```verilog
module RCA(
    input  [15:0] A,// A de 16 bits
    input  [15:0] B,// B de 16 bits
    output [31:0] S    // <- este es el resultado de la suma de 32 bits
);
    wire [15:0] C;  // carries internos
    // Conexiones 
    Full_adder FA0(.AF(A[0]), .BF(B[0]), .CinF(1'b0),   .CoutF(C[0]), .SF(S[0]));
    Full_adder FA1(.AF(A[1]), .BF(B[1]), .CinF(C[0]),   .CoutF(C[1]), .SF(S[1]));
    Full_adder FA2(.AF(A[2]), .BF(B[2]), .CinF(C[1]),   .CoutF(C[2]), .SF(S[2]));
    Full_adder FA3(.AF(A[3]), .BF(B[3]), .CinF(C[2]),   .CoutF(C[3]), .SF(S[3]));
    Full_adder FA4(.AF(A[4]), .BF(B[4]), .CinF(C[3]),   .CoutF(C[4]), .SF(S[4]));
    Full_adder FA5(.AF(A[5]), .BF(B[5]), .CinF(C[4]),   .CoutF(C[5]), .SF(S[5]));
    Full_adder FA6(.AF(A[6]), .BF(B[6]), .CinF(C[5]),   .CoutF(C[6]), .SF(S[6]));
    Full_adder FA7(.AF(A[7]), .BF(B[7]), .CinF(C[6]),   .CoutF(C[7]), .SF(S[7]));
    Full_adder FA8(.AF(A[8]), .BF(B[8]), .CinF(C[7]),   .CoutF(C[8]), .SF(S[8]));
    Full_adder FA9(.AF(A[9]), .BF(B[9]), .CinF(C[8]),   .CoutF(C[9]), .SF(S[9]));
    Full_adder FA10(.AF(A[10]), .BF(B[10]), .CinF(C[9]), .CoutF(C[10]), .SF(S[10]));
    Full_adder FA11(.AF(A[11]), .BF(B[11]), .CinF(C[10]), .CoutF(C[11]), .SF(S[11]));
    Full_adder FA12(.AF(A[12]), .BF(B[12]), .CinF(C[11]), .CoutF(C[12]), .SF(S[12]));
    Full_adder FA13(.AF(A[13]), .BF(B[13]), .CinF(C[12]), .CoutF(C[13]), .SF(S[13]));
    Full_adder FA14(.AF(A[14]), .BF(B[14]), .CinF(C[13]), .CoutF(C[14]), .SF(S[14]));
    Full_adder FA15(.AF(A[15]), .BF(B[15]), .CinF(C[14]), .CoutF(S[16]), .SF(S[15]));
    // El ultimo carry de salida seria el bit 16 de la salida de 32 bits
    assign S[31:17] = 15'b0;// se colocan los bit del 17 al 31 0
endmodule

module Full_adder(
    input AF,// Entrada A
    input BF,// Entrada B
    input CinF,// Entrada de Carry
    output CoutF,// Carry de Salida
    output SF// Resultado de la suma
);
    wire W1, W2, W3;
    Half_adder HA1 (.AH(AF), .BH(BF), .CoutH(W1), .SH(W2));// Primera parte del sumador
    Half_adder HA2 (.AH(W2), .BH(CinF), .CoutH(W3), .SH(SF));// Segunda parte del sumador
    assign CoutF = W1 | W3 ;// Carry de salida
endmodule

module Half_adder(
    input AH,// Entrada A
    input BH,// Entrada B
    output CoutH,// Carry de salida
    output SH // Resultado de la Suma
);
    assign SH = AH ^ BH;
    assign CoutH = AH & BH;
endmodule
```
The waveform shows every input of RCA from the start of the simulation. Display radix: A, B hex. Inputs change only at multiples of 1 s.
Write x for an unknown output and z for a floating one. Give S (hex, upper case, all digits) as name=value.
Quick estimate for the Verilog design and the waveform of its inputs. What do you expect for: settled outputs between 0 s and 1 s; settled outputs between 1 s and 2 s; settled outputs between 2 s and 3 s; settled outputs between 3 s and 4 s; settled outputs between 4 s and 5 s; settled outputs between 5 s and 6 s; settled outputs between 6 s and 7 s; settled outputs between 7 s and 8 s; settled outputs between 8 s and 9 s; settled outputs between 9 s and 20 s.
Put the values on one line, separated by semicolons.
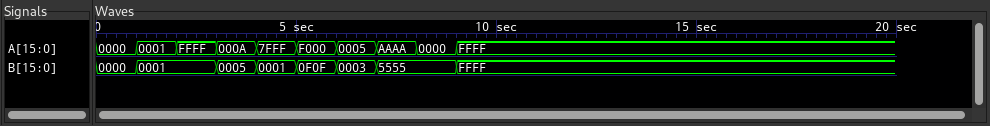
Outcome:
S=00000000; S=00000002; S=00010000; S=0000000F; S=00008000; S=0000FF0F; S=00000008; S=0000FFFF; S=00005555; S=0001FFFE
